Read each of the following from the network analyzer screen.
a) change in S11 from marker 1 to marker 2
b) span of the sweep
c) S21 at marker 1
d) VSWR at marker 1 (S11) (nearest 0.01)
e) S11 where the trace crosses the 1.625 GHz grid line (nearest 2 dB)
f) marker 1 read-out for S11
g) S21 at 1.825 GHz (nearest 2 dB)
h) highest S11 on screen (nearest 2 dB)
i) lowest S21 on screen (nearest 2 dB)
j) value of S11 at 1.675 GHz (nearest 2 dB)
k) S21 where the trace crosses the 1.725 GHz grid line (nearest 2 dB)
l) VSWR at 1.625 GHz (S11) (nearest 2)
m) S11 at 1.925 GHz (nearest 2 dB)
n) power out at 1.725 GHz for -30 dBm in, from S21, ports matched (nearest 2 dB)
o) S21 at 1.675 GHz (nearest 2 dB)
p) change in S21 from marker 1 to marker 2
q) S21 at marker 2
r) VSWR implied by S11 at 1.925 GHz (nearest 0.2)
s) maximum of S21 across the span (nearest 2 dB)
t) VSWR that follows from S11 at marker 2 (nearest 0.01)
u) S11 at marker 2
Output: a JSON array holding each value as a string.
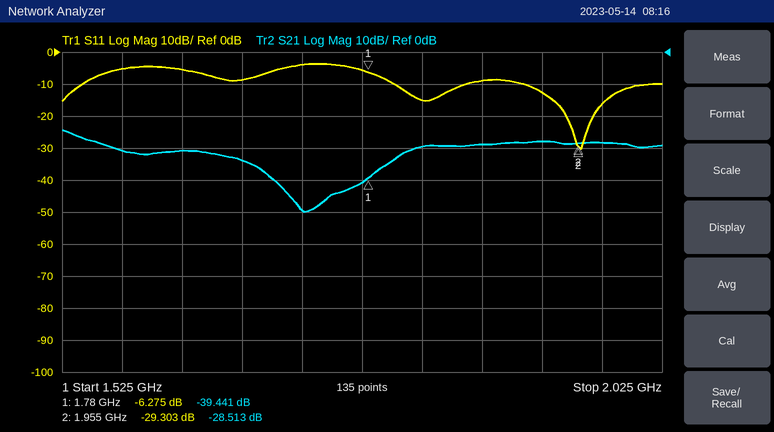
["-23.028 dB", "500 MHz", "-39.441 dB", "2.89", "-6 dB", "-6.275 dB", "-30 dB", "-4 dB", "-50 dB", "-8 dB", "-50 dB", "4", "-12 dB", "-80 dBm", "-34 dB", "10.928 dB", "-28.513 dB", "1.6", "-24 dB", "1.07", "-29.303 dB"]
